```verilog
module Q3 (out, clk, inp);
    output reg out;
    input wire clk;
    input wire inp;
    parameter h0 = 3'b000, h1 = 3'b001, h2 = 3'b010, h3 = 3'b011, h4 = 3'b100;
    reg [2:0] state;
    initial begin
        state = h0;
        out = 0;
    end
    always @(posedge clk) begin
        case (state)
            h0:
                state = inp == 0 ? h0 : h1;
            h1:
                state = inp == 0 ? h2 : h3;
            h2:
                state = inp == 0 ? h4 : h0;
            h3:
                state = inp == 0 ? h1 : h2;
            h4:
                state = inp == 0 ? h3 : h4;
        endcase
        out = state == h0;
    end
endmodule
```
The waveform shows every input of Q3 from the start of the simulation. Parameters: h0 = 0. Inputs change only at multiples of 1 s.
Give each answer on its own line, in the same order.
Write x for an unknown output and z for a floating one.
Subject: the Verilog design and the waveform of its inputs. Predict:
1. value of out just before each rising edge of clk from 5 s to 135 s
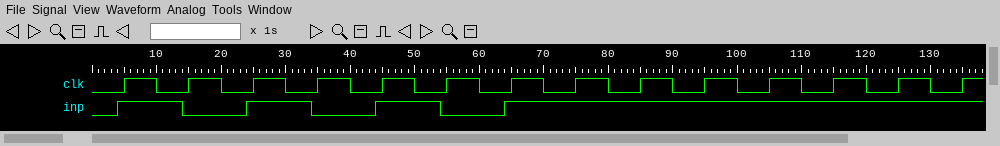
0 0 0 1 1 0 0 1 0 0 0 1 0 0
